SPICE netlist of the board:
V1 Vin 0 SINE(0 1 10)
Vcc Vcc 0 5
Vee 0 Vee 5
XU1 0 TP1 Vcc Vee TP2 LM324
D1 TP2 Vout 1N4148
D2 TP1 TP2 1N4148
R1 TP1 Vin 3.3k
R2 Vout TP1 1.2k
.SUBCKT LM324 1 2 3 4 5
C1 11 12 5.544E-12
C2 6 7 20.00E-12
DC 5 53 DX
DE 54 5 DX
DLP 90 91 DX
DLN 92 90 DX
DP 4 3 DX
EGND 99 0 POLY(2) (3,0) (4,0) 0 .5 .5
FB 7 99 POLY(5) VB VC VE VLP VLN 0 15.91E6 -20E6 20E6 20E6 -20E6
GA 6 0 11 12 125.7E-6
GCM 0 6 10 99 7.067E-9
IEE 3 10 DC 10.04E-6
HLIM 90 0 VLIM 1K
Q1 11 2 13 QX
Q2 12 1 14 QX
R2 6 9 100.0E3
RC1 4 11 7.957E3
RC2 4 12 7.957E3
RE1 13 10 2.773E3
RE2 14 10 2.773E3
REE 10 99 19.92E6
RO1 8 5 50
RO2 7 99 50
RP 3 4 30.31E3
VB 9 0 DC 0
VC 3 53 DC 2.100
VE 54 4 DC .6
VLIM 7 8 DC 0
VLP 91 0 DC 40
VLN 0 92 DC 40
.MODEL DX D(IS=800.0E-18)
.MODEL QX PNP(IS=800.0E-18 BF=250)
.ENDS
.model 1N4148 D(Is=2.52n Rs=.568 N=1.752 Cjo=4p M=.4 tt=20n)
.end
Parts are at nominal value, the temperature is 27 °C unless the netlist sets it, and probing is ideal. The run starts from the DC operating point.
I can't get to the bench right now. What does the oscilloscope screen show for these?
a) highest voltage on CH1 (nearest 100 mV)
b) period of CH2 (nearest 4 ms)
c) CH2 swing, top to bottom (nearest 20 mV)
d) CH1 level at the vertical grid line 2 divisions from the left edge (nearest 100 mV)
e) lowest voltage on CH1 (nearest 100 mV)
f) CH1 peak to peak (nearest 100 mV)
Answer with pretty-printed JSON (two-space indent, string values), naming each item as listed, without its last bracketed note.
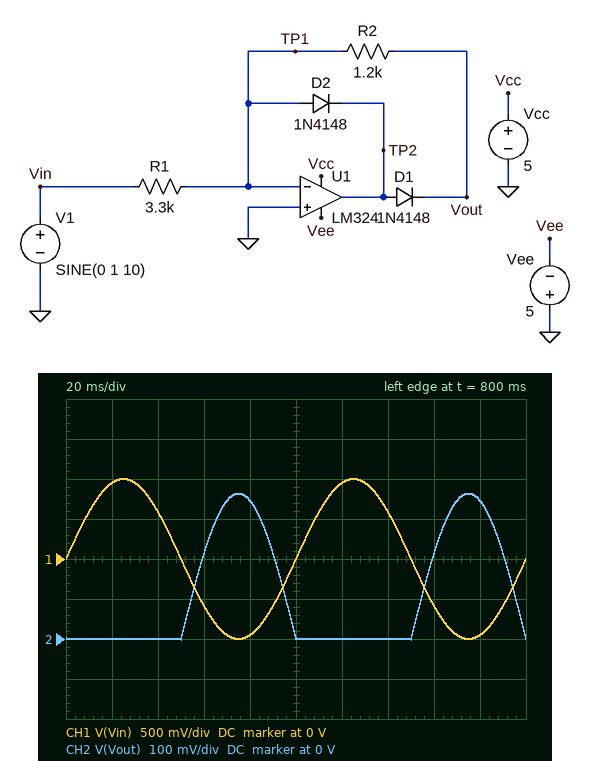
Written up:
{
  "highest voltage on CH1": "1.0 V",
  "period of CH2": "100 ms",
  "CH2 swing, top to bottom": "360 mV",
  "CH1 level at the vertical grid line 2 divisions from the left edge": "600 mV",
  "lowest voltage on CH1": "-1.0 V",
  "CH1 peak to peak": "2.0 V"
}
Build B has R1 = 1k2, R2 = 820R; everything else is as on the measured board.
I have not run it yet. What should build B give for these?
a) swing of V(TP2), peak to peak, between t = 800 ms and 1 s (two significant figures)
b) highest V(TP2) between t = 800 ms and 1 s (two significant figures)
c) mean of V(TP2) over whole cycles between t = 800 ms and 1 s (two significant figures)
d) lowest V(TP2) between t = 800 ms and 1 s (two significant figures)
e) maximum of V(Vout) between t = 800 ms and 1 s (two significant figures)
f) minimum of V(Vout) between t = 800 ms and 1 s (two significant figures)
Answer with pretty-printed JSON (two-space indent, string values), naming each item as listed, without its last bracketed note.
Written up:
{
  "swing of V(TP2), peak to peak, between t = 800 ms and 1 s": "1.8 V",
  "highest V(TP2) between t = 800 ms and 1 s": "1.3 V",
  "mean of V(TP2) over whole cycles between t = 800 ms and 1 s": "220 mV",
  "lowest V(TP2) between t = 800 ms and 1 s": "-580 mV",
  "maximum of V(Vout) between t = 800 ms and 1 s": "680 mV",
  "minimum of V(Vout) between t = 800 ms and 1 s": "-2.4 mV"
}
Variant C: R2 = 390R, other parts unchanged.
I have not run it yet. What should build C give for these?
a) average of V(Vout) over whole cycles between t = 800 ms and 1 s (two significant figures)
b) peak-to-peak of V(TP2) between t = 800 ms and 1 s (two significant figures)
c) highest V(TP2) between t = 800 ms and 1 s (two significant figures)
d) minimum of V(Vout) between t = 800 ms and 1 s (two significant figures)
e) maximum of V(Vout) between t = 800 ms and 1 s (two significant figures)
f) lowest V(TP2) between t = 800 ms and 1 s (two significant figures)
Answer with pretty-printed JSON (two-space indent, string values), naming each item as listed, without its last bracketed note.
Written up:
{
  "average of V(Vout) over whole cycles between t = 800 ms and 1 s": "38 mV",
  "peak-to-peak of V(TP2) between t = 800 ms and 1 s": "1.2 V",
  "highest V(TP2) between t = 800 ms and 1 s": "650 mV",
  "minimum of V(Vout) between t = 800 ms and 1 s": "-2.1 mV",
  "maximum of V(Vout) between t = 800 ms and 1 s": "120 mV",
  "lowest V(TP2) between t = 800 ms and 1 s": "-530 mV"
}
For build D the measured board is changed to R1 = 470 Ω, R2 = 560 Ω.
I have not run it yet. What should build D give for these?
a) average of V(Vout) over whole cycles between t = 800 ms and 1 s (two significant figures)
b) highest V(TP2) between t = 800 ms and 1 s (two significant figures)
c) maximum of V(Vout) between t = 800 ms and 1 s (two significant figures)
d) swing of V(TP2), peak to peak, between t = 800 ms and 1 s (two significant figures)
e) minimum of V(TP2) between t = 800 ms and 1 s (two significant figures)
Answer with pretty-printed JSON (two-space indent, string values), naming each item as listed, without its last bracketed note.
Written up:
{
  "average of V(Vout) over whole cycles between t = 800 ms and 1 s": "380 mV",
  "highest V(TP2) between t = 800 ms and 1 s": "1.8 V",
  "maximum of V(Vout) between t = 800 ms and 1 s": "1.2 V",
  "swing of V(TP2), peak to peak, between t = 800 ms and 1 s": "2.4 V",
  "minimum of V(TP2) between t = 800 ms and 1 s": "-620 mV"
}
